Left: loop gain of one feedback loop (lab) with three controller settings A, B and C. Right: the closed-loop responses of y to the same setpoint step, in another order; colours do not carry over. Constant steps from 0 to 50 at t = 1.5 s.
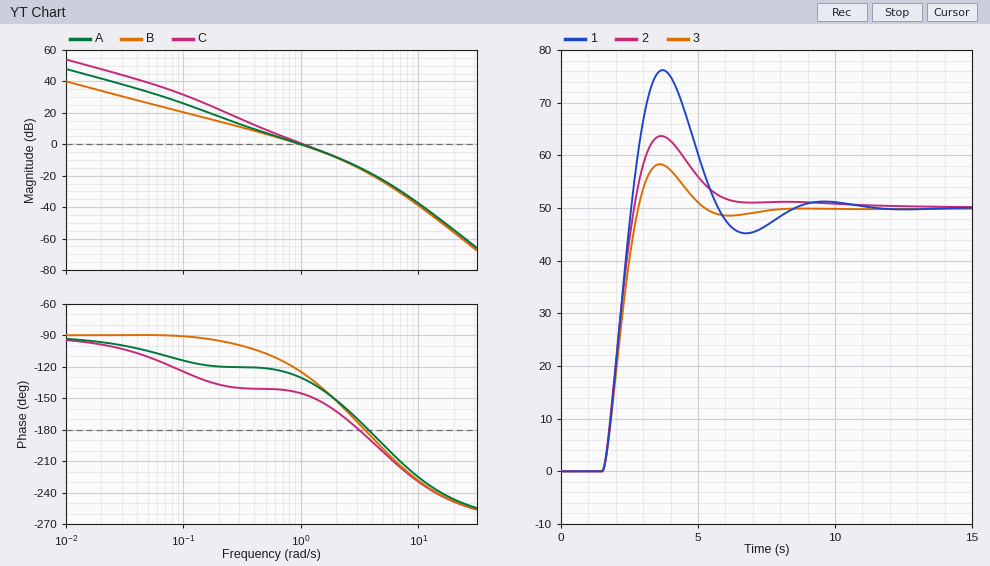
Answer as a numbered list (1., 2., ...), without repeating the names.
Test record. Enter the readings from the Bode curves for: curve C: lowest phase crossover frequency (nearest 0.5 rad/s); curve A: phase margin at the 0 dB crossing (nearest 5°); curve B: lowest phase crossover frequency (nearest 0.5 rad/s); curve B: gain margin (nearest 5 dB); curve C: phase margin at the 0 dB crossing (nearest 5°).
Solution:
1. 3.0 rad/s
2. 50°
3. 3.5 rad/s
4. 15 dB
5. 35°
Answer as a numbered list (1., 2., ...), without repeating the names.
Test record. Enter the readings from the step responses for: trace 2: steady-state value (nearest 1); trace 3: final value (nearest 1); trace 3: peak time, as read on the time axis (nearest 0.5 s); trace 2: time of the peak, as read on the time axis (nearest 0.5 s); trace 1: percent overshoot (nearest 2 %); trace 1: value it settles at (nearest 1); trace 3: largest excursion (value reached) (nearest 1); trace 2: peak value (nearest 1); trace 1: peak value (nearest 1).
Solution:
1. 50
2. 50
3. 3.5 s
4. 3.5 s
5. 52 %
6. 50
7. 58
8. 64
9. 76
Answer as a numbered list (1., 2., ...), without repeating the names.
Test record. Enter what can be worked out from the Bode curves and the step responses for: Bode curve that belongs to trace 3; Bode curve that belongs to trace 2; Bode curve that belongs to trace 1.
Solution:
1. B
2. A
3. C
